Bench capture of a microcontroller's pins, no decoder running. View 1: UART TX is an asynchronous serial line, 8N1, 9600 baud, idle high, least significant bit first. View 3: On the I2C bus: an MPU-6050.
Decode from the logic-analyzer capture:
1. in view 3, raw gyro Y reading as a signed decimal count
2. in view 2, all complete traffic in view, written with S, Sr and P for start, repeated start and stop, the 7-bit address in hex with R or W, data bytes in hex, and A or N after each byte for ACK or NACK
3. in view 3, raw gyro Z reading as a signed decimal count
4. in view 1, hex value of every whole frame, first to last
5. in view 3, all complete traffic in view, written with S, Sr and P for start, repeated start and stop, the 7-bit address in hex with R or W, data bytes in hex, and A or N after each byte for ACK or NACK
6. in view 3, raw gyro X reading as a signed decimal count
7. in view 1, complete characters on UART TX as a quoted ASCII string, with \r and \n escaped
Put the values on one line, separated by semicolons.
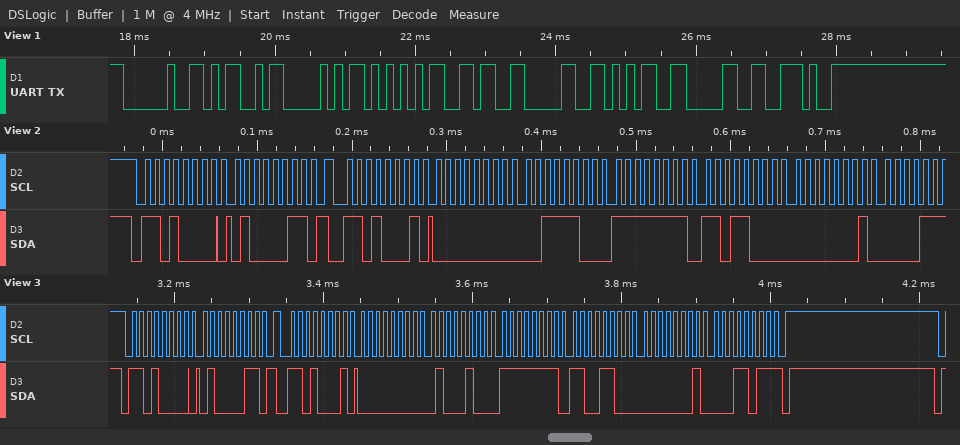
-52; S 68W A 43 A Sr 68R A 00 A 3C A FF A D8 A 01 A; 283; 0x20 0x4D 0x50 0x55 0x36 0x30 0x35 0x30 0x2E; S 68W A 43 A Sr 68R A 00 A 44 A FF A CC A 01 A 1B N P; 68; " MPU6050."
